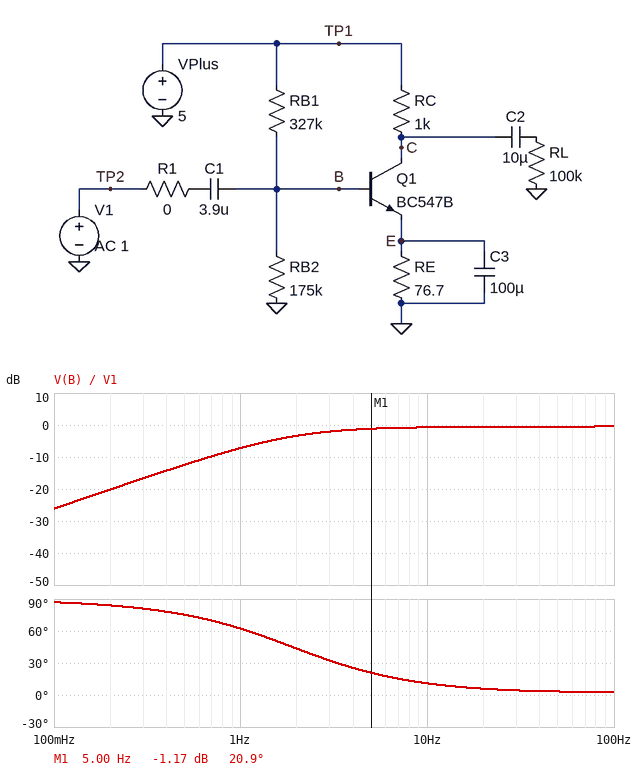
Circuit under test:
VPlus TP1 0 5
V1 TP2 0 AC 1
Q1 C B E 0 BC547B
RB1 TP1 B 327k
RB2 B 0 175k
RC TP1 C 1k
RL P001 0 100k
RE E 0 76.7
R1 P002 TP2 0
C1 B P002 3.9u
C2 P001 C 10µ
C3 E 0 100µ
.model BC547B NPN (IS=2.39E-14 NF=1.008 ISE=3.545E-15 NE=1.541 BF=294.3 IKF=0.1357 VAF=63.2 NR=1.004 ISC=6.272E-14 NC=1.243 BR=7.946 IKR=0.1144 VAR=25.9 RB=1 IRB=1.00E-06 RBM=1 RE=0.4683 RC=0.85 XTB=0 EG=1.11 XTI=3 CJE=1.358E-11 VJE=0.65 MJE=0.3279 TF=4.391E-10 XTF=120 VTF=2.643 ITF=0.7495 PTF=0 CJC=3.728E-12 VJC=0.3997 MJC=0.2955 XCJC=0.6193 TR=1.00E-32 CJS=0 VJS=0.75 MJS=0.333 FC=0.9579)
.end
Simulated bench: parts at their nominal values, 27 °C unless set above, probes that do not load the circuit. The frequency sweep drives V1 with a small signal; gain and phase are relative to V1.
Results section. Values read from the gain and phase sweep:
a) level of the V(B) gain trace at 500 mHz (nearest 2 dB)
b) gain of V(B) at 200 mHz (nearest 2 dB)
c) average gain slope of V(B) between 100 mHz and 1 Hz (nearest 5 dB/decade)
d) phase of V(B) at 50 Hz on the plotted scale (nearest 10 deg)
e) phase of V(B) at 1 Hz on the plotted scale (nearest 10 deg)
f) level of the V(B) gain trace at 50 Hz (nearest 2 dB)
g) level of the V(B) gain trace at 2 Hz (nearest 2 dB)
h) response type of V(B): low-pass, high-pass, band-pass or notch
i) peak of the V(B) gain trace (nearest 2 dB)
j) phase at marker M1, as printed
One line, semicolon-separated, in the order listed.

-12 dB; -20 dB; 20 dB/decade; 0 deg; 60 deg; 0 dB; -4 dB; high-pass; 0 dB; 20.9 deg
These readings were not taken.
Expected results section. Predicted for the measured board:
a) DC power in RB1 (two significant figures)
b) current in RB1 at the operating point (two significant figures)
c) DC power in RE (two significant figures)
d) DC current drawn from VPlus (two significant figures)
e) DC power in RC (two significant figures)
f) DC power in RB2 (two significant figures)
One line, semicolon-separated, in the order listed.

53 µW; 13 µA; 410 µW; 2.3 mA; 5.3 mW; 4.0 µW
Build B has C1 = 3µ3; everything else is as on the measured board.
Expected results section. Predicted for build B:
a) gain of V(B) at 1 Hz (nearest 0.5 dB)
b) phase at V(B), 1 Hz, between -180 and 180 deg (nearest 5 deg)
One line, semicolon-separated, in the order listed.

-8.5 dB; 65 deg
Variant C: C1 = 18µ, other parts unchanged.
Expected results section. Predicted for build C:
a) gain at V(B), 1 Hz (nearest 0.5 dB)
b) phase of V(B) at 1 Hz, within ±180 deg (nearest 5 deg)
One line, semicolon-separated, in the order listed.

-1.0 dB; 25 deg
